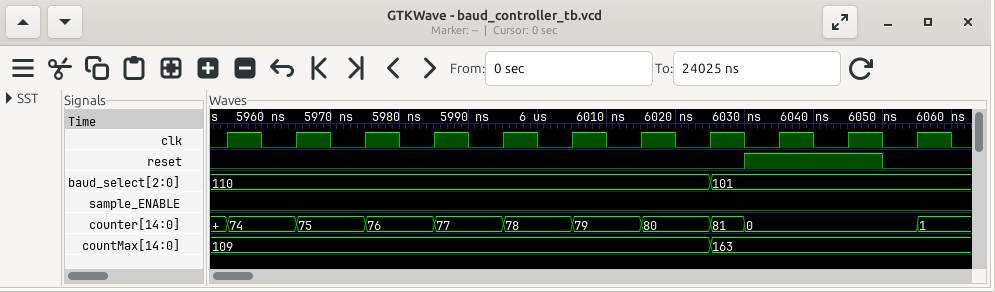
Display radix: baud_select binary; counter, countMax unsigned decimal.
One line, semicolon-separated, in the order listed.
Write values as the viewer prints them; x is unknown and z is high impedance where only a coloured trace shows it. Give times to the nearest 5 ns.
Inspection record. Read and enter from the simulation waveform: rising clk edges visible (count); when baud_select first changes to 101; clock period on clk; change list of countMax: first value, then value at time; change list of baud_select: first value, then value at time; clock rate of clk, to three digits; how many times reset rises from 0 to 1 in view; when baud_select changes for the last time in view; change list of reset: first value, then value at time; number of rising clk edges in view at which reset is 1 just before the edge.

11; 6025 ns; 10 ns; 109, 163 at 6025 ns; 110, 101 at 6025 ns; 100 MHz; 1; 6025 ns; 0, 1 at 6030 ns, 0 at 6050 ns; 2
